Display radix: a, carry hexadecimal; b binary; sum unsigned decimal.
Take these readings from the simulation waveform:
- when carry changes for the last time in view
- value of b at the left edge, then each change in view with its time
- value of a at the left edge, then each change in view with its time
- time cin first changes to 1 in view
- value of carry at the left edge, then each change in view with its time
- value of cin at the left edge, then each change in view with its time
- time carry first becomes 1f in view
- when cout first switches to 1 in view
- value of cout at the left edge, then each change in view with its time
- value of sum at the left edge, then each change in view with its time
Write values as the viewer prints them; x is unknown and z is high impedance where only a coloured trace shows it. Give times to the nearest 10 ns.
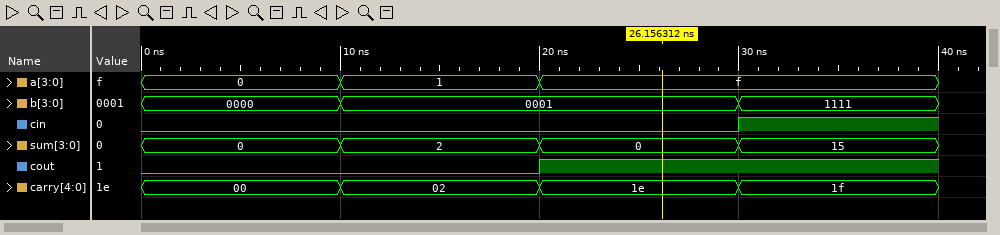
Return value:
30 ns
0000, 0001 at 10 ns, 1111 at 30 ns
0, 1 at 10 ns, f at 20 ns
30 ns
00, 02 at 10 ns, 1e at 20 ns, 1f at 30 ns
0, 1 at 30 ns
30 ns
20 ns
0, 1 at 20 ns
0, 2 at 10 ns, 0 at 20 ns, 15 at 30 ns
